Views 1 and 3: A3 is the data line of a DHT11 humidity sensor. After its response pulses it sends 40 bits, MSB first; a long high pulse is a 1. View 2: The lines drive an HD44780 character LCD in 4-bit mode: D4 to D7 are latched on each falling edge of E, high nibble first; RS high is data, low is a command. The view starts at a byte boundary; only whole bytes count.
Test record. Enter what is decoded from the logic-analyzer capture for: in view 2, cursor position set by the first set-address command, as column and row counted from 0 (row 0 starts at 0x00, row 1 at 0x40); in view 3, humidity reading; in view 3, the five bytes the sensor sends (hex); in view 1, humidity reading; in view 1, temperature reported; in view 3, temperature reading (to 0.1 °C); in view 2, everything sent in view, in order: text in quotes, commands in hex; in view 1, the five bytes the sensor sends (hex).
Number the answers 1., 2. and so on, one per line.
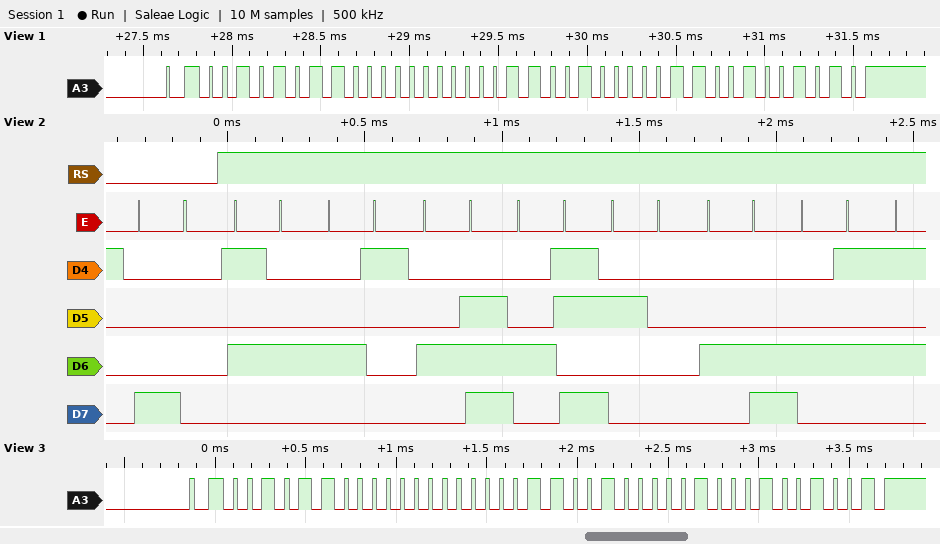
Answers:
1. column 0, row 0
2. 44 %
3. 2C 00 19 04 49
4. 43 %
5. 25.6 °C
6. 25.4 °C
7. 0x80 "TANK LE"
8. 2B 00 19 06 4A
